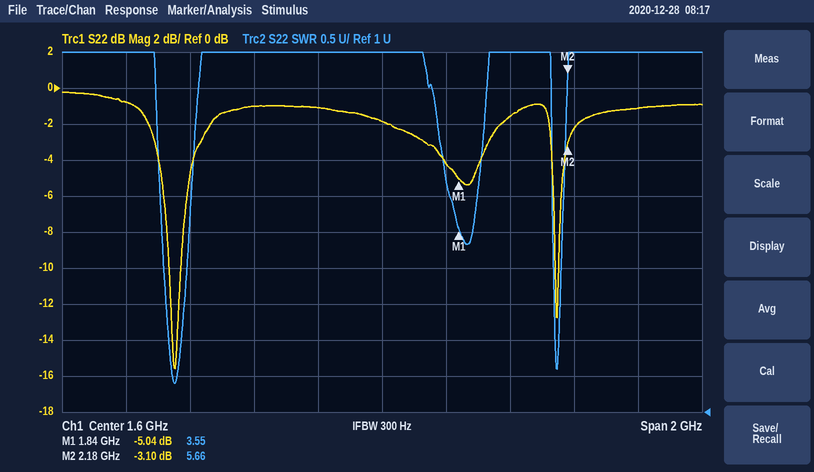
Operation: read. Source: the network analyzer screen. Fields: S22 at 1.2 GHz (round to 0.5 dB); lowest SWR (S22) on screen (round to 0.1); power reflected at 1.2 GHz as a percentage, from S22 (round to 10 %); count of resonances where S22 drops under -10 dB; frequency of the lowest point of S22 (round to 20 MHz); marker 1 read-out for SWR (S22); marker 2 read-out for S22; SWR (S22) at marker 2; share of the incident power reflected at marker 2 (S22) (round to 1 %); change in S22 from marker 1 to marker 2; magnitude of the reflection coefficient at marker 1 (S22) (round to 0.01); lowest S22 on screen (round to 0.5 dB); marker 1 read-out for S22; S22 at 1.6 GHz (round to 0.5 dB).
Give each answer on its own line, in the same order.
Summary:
-1.0 dB
1.4
80 %
2
960 MHz
3.55
-3.10 dB
5.66
49 %
1.94 dB
0.56
-15.5 dB
-5.04 dB
-2.0 dB
